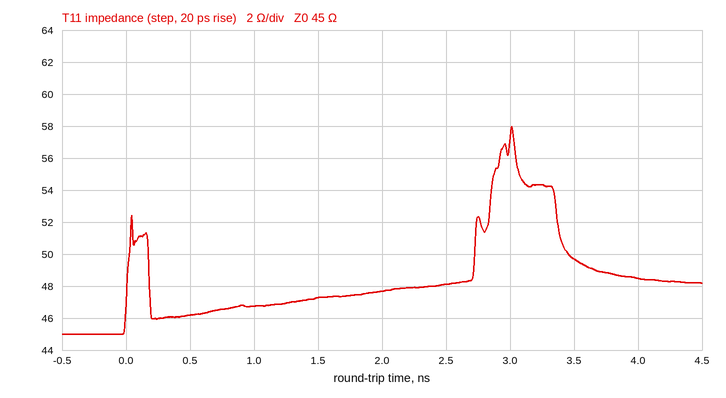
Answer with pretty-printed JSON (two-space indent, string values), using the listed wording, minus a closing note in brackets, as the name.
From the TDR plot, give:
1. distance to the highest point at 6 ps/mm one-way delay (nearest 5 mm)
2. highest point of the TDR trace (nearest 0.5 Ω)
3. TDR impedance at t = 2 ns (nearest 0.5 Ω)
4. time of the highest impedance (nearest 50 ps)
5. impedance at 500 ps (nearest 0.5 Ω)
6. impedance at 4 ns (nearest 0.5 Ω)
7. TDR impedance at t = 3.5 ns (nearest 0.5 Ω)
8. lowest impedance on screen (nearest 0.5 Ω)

{
  "distance to the highest point at 6 ps/mm one-way delay": "250 mm",
  "highest point of the TDR trace": "58.0 Ω",
  "TDR impedance at t = 2 ns": "47.5 Ω",
  "time of the highest impedance": "3.00 ns",
  "impedance at 500 ps": "46.0 Ω",
  "impedance at 4 ns": "48.5 Ω",
  "TDR impedance at t = 3.5 ns": "49.5 Ω",
  "lowest impedance on screen": "45.0 Ω"
}
